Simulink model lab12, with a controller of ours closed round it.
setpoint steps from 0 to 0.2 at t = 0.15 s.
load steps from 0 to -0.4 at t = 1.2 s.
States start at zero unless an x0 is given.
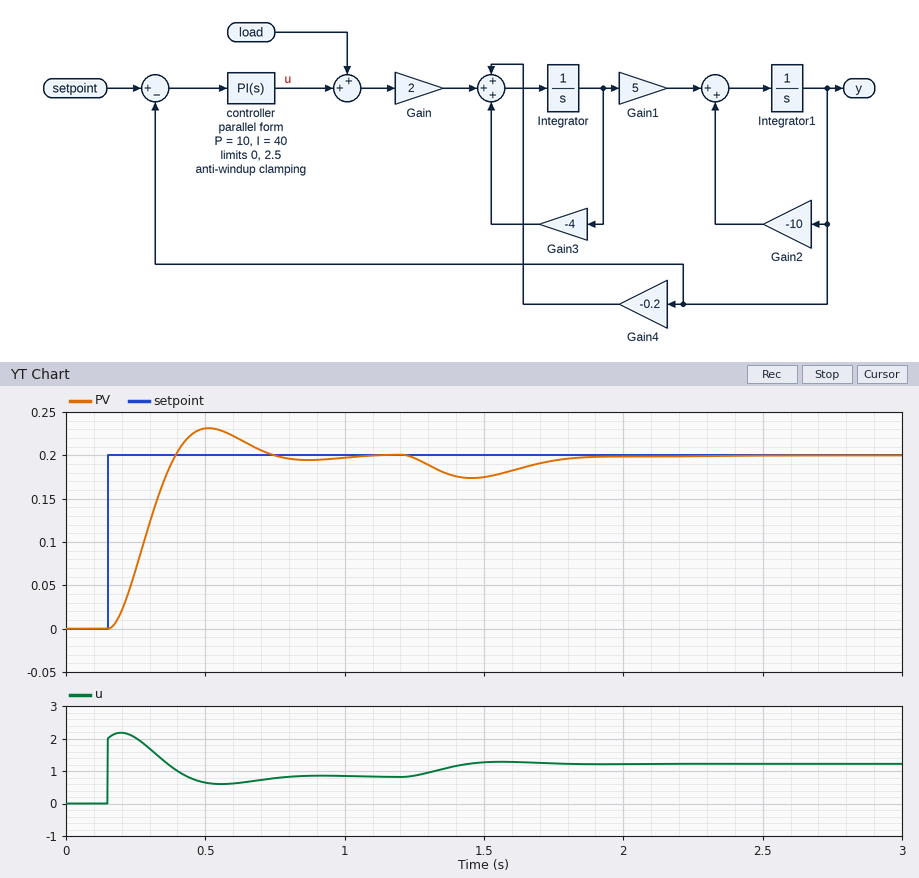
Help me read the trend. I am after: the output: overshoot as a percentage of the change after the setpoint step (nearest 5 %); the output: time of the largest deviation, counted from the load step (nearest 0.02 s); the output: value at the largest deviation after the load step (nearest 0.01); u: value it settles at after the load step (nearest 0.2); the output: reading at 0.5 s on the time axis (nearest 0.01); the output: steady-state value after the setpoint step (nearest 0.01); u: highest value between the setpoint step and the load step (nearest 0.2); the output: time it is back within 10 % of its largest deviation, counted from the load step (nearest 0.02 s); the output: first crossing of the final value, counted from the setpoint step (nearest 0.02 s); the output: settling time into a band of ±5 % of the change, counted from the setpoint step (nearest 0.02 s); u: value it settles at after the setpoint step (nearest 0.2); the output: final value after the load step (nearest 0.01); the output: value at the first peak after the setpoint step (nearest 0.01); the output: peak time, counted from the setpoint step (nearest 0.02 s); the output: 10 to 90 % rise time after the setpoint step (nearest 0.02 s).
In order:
15 %
0.26 s
0.17
1.2
0.23
0.20
2.2
0.64 s
0.24 s
0.52 s
0.8
0.20
0.23
0.36 s
0.16 s
